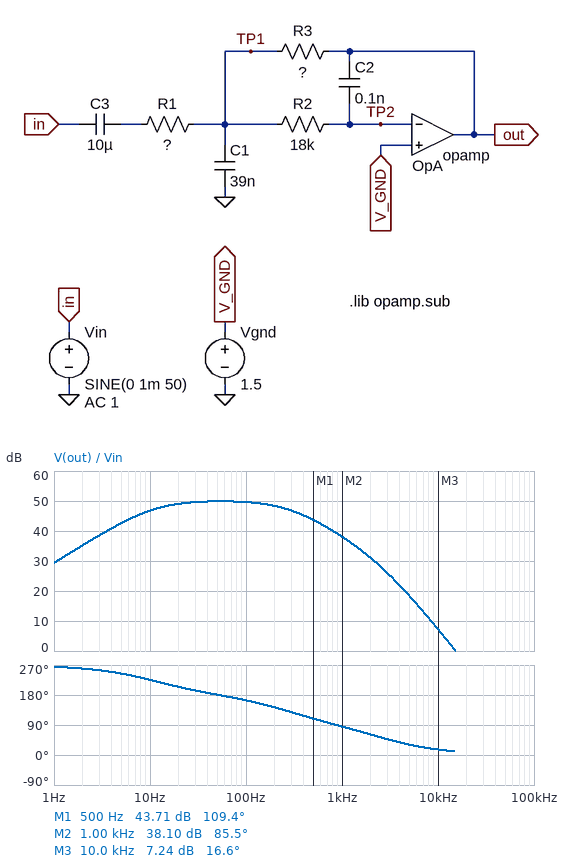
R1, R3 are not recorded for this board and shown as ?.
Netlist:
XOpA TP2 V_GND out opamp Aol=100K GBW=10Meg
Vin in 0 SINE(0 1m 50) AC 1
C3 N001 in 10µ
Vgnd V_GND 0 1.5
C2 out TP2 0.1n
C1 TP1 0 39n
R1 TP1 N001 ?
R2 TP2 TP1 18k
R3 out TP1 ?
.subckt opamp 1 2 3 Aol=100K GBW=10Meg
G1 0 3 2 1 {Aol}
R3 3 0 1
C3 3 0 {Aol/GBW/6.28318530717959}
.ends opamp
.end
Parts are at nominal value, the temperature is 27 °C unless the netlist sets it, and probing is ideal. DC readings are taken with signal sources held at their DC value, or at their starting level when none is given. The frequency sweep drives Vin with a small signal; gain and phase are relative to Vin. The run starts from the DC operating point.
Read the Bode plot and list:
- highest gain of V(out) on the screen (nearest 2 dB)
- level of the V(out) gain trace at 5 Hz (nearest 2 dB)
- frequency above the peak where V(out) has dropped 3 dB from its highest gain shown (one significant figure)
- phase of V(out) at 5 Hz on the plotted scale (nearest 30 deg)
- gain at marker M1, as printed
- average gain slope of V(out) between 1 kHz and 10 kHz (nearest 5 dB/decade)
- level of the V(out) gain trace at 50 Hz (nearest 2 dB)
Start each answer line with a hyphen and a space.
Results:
- 50 dB
- 42 dB
- 300 Hz
- 240 deg
- 43.71 dB
- -30 dB/decade
- 50 dB
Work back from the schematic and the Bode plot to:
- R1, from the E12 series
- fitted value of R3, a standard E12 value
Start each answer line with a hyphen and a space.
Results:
- 1.5 kΩ
- 470 kΩ
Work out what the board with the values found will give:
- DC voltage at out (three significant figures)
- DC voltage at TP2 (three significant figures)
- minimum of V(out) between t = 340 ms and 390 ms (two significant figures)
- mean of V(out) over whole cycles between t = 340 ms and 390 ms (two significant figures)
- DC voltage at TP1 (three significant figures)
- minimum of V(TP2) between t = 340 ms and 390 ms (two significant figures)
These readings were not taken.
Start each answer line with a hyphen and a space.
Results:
- 1.50 V
- 1.50 V
- 1.2 V
- 1.5 V
- 1.50 V
- 1.5 V
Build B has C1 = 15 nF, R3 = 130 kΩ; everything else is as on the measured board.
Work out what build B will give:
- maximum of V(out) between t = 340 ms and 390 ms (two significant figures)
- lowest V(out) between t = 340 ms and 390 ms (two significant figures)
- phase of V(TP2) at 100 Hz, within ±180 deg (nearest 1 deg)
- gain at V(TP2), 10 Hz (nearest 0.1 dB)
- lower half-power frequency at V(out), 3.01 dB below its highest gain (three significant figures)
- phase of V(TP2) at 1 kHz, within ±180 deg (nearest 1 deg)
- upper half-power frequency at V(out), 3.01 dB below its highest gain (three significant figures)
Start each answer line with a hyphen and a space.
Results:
- 1.6 V
- 1.4 V
- 45 deg
- -64.4 dB
- 10.5 Hz
- 33 deg
- 1.06 kHz
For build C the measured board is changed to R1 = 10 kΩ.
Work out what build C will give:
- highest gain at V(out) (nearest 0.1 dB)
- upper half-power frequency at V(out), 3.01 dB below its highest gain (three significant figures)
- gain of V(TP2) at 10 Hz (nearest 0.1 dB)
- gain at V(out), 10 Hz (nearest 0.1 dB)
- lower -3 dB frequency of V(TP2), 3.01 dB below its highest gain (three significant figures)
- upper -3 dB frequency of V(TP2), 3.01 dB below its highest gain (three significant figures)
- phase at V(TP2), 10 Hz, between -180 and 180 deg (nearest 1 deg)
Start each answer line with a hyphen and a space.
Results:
- 36.7 dB
- 1.04 kHz
- -66.6 dB
- 33.3 dB
- 605 Hz
- 1.25 kHz
- 14 deg
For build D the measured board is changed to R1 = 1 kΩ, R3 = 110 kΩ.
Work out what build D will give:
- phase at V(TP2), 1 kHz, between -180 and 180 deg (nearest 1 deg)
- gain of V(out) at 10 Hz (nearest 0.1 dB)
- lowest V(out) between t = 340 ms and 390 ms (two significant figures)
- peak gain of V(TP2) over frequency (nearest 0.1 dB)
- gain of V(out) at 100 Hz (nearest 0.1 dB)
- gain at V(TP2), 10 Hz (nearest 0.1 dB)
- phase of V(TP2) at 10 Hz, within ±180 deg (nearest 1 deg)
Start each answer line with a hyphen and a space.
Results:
- 22 deg
- 35.4 dB
- 1.4 V
- -41.7 dB
- 40.8 dB
- -64.6 dB
- 63 deg
